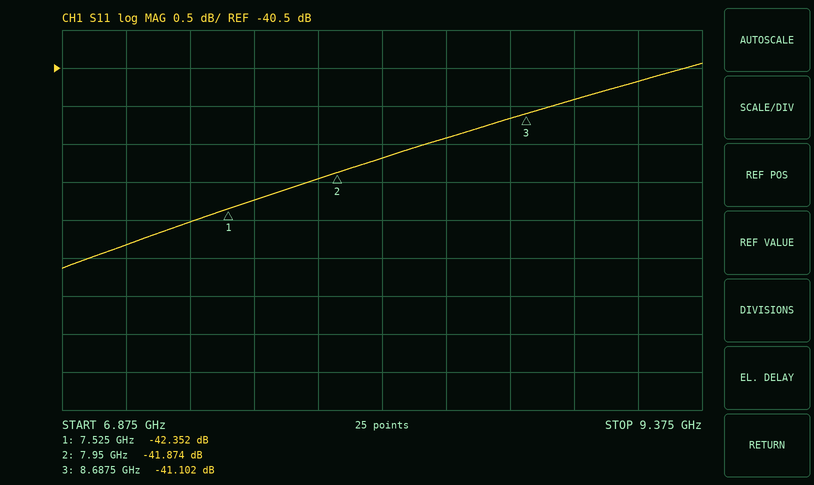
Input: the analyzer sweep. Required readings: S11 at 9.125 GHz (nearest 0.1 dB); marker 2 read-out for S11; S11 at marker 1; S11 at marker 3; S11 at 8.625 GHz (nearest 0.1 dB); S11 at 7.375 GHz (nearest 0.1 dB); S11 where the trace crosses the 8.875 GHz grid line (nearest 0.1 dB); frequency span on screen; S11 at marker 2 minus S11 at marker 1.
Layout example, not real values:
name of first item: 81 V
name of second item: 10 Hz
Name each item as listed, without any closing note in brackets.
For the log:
S11 at 9.125 GHz: -40.7 dB
marker 2 read-out for S11: -41.874 dB
S11 at marker 1: -42.352 dB
S11 at marker 3: -41.102 dB
S11 at 8.625 GHz: -41.2 dB
S11 at 7.375 GHz: -42.5 dB
S11 where the trace crosses the 8.875 GHz grid line: -40.9 dB
frequency span on screen: 2.5 GHz
S11 at marker 2 minus S11 at marker 1: 0.478 dB
